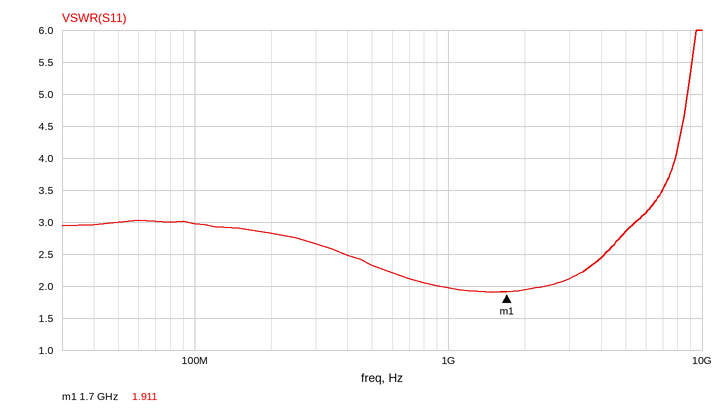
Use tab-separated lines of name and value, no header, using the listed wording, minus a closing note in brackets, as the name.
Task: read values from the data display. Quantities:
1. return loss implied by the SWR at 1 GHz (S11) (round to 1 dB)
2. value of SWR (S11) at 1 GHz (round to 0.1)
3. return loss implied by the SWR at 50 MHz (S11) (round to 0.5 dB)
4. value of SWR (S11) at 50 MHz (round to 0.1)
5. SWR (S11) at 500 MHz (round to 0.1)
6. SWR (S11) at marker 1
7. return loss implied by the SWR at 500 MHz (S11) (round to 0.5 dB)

return loss implied by the SWR at 1 GHz (S11)	10 dB
value of SWR (S11) at 1 GHz	2.0
return loss implied by the SWR at 50 MHz (S11)	6.0 dB
value of SWR (S11) at 50 MHz	3.0
SWR (S11) at 500 MHz	2.3
SWR (S11) at marker 1	1.911
return loss implied by the SWR at 500 MHz (S11)	8.0 dB
